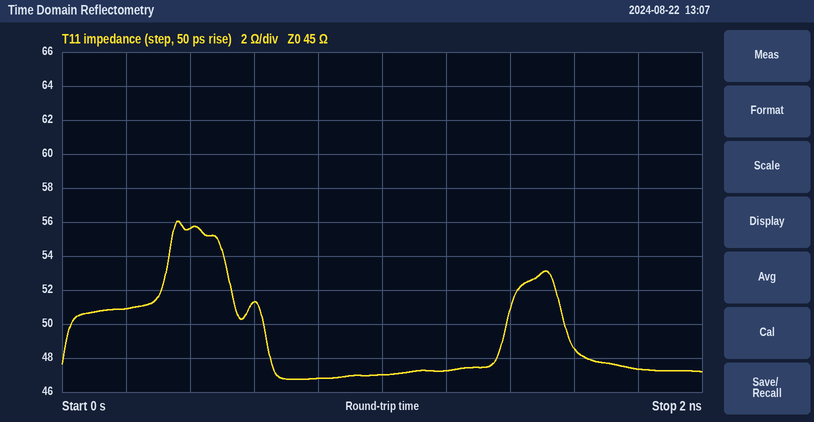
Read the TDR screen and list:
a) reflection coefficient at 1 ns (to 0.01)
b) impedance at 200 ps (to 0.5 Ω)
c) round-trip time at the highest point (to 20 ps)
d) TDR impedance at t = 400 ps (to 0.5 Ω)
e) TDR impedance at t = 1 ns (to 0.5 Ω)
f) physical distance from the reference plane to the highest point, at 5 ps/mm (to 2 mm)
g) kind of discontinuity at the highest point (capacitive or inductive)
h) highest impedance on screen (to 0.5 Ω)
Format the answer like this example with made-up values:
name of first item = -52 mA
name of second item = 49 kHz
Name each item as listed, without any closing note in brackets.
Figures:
reflection coefficient at 1 ns = +0.02
impedance at 200 ps = 51.0 Ω
round-trip time at the highest point = 360 ps
TDR impedance at t = 400 ps = 55.5 Ω
TDR impedance at t = 1 ns = 47.0 Ω
physical distance from the reference plane to the highest point, at 5 ps/mm = 36 mm
kind of discontinuity at the highest point = inductive
highest impedance on screen = 56.0 Ω
